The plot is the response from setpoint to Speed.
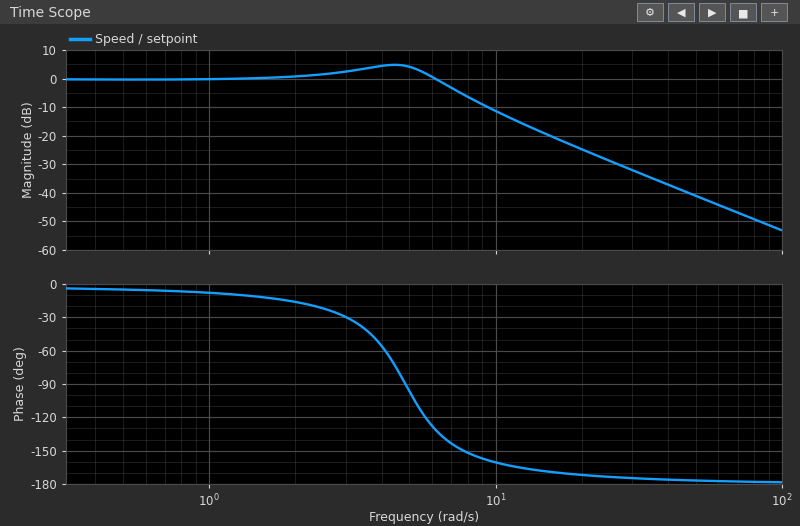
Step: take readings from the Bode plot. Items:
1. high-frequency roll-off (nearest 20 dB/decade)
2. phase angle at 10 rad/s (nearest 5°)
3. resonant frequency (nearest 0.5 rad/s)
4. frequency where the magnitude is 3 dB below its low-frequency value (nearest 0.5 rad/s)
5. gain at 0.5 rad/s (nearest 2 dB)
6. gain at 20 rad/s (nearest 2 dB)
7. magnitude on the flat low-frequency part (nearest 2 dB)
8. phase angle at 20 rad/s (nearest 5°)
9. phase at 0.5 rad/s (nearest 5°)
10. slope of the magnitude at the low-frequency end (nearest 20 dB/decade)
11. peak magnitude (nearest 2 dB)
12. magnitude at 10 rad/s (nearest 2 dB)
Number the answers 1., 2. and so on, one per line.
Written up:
1. -40 dB/decade
2. -160°
3. 4.5 rad/s
4. 7.0 rad/s
5. 0 dB
6. -24 dB
7. 0 dB
8. -170°
9. -5°
10. 0 dB/decade
11. 4 dB
12. -12 dB
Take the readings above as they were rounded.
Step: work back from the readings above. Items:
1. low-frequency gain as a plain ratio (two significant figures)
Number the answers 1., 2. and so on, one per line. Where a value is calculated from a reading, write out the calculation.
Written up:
1. 10^(0 / 20) = 1.0
